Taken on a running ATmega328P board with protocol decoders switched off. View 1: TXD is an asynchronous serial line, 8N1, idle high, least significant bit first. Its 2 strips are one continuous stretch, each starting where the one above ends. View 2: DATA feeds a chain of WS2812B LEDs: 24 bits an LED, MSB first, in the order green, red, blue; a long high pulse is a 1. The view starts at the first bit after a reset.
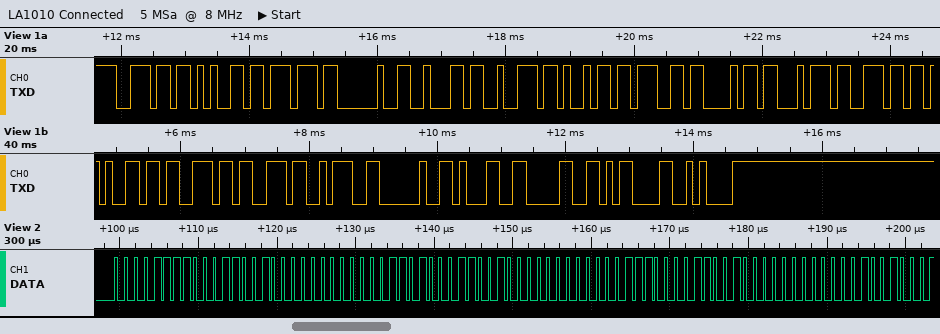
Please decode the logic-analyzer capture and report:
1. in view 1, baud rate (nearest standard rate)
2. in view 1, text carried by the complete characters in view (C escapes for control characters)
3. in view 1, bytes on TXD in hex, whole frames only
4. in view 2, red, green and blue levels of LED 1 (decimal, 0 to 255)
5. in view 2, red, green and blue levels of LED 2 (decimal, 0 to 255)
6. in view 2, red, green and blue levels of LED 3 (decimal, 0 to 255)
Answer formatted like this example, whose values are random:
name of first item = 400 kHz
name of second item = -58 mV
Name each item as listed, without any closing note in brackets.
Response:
in view 1, baud rate = 9600 baud
in view 1, text carried by the complete characters in view = "new brightness: 10\r\n"
in view 1, bytes on TXD in hex, whole frames only = 6E 65 77 20 62 72 69 67 68 74 6E 65 73 73 3A 20 31 30 0D 0A
in view 2, red, green and blue levels of LED 1 = 25, 15, 0
in view 2, red, green and blue levels of LED 2 = 25, 13, 0
in view 2, red, green and blue levels of LED 3 = 25, 14, 0
